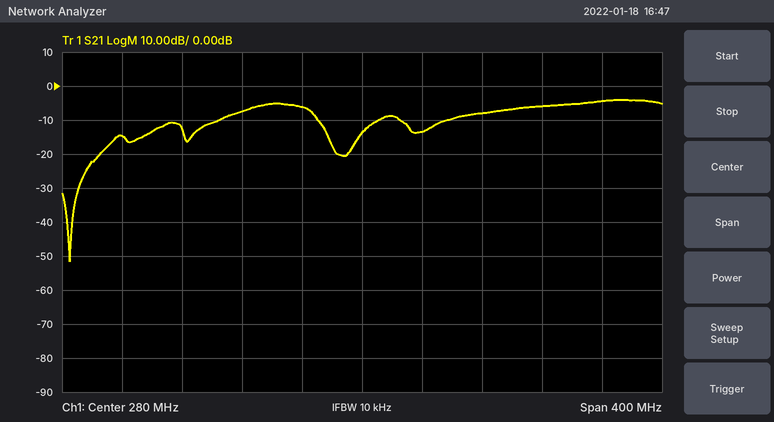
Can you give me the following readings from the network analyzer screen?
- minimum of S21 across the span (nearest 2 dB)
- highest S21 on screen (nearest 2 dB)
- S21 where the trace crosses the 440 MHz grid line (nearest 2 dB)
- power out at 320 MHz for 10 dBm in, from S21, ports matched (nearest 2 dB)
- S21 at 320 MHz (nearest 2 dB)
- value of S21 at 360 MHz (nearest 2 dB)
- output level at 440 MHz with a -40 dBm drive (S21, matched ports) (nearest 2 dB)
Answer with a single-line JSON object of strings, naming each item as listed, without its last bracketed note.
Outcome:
{"minimum of S21 across the span": "-52 dB", "highest S21 on screen": "-4 dB", "S21 where the trace crosses the 440 MHz grid line": "-4 dB", "power out at 320 MHz for 10 dBm in, from S21, ports matched": "-4 dBm", "S21 at 320 MHz": "-14 dB", "value of S21 at 360 MHz": "-8 dB", "output level at 440 MHz with a -40 dBm drive (S21, matched ports)": "-44 dBm"}
